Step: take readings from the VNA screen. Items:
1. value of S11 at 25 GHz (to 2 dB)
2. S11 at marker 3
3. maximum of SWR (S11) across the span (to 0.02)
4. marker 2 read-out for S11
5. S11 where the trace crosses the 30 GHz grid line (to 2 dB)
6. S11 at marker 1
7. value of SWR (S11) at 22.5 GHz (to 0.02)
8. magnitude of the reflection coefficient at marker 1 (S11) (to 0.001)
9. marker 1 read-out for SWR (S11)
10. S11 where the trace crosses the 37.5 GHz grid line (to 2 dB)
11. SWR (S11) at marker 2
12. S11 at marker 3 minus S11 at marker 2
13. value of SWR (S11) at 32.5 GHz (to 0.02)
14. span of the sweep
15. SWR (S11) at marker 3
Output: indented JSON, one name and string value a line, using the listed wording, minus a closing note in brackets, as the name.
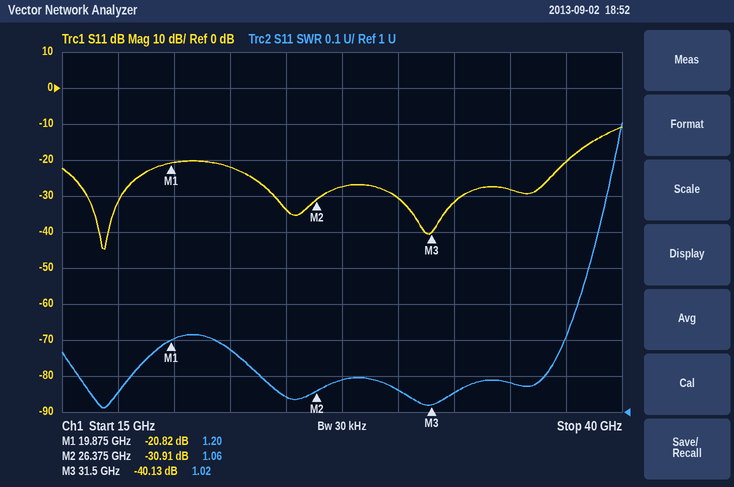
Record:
{
  "value of S11 at 25 GHz": "-34 dB",
  "S11 at marker 3": "-40.13 dB",
  "maximum of SWR (S11) across the span": "1.80",
  "marker 2 read-out for S11": "-30.91 dB",
  "S11 where the trace crosses the 30 GHz grid line": "-30 dB",
  "S11 at marker 1": "-20.82 dB",
  "value of SWR (S11) at 22.5 GHz": "1.18",
  "magnitude of the reflection coefficient at marker 1 (S11)": "0.091",
  "marker 1 read-out for SWR": "1.20",
  "S11 where the trace crosses the 37.5 GHz grid line": "-20 dB",
  "SWR (S11) at marker 2": "1.06",
  "S11 at marker 3 minus S11 at marker 2": "-9.22 dB",
  "value of SWR (S11) at 32.5 GHz": "1.06",
  "span of the sweep": "25 GHz",
  "SWR (S11) at marker 3": "1.02"
}
